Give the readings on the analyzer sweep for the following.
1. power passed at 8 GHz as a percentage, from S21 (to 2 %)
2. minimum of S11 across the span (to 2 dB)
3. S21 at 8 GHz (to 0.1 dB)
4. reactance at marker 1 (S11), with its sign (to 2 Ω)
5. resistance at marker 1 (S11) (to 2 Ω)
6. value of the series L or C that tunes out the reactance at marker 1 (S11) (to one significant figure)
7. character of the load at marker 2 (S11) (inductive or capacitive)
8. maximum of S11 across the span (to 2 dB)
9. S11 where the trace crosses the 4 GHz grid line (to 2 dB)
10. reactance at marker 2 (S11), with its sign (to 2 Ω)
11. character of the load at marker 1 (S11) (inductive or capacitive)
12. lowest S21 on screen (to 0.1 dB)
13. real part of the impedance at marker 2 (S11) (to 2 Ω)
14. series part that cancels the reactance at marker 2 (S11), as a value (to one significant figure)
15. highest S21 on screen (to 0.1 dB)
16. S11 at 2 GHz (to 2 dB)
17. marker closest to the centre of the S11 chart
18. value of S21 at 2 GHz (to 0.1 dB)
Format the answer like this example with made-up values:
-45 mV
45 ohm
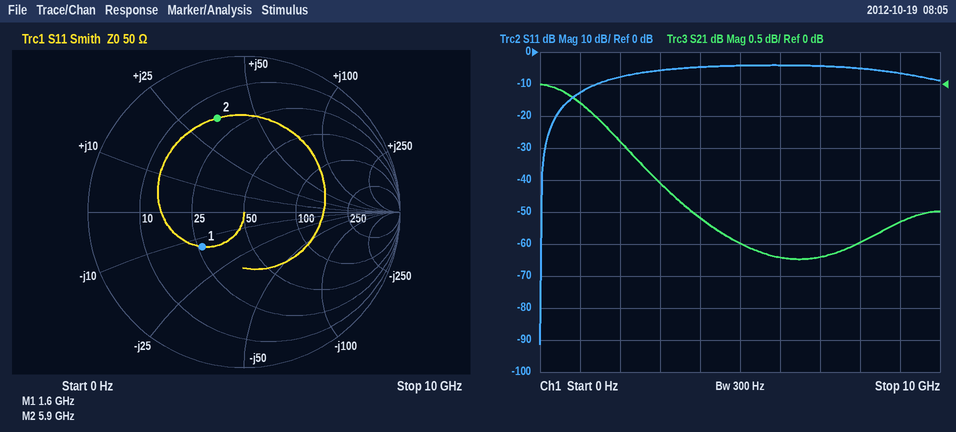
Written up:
56 %
-92 dB
-2.5 dB
-14 Ω
26 Ω
1 nH
inductive
-4 dB
-4 dB
+34 Ω
capacitive
-2.7 dB
18 Ω
800 fF
0.0 dB
-8 dB
marker 1
-0.9 dB
